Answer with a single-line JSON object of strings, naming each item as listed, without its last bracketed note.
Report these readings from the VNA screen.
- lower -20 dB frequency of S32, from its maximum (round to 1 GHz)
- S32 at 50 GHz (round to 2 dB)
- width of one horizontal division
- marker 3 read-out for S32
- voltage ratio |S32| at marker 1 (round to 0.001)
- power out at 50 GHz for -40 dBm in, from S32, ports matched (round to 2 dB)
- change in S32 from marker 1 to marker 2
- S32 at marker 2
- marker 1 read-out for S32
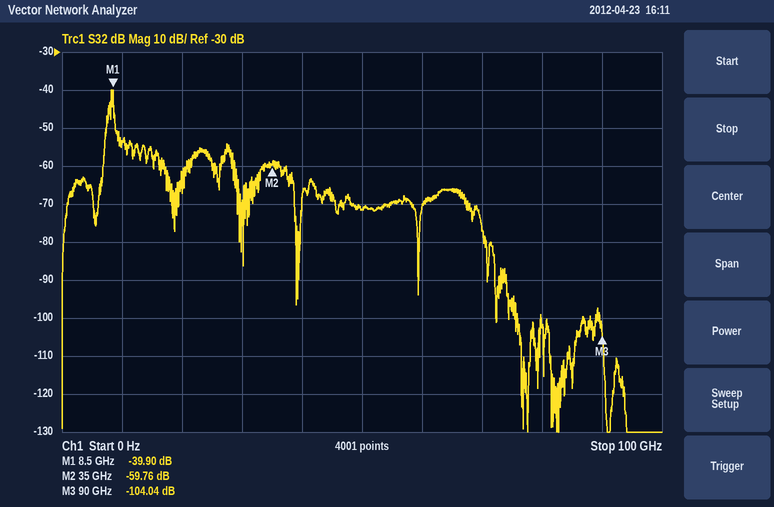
{"lower -20 dB frequency of S32, from its maximum": "7 GHz", "S32 at 50 GHz": "-72 dB", "width of one horizontal division": "10 GHz", "marker 3 read-out for S32": "-104.04 dB", "voltage ratio |S32| at marker 1": "0.010", "power out at 50 GHz for -40 dBm in, from S32, ports matched": "-112 dBm", "change in S32 from marker 1 to marker 2": "-19.86 dB", "S32 at marker 2": "-59.76 dB", "marker 1 read-out for S32": "-39.90 dB"}
